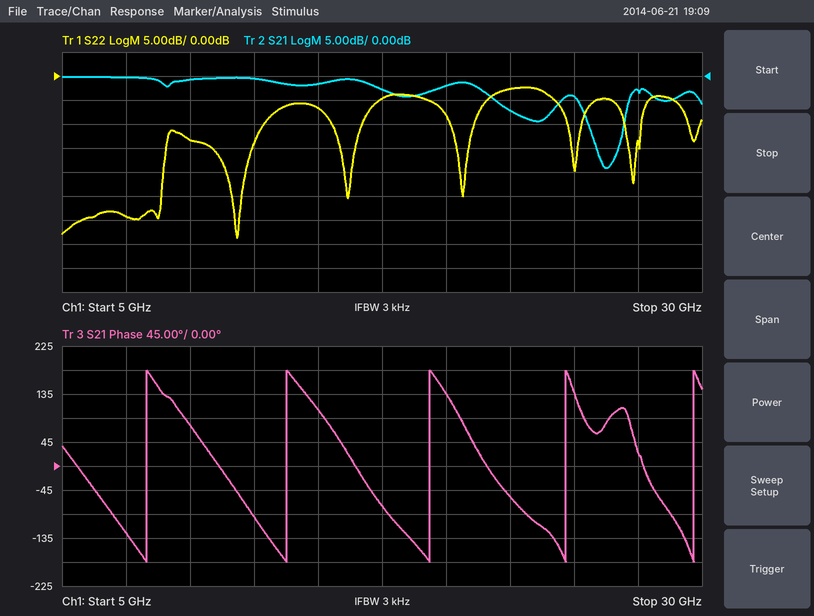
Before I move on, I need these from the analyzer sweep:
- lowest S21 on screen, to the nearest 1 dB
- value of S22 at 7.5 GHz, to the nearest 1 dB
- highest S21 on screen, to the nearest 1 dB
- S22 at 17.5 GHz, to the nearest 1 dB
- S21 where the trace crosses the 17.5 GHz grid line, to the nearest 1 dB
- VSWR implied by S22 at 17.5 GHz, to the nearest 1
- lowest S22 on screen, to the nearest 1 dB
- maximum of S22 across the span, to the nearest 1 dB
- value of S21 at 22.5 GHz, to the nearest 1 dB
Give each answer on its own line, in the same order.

-19 dB
-29 dB
0 dB
-5 dB
-3 dB
4
-34 dB
-2 dB
-7 dB
